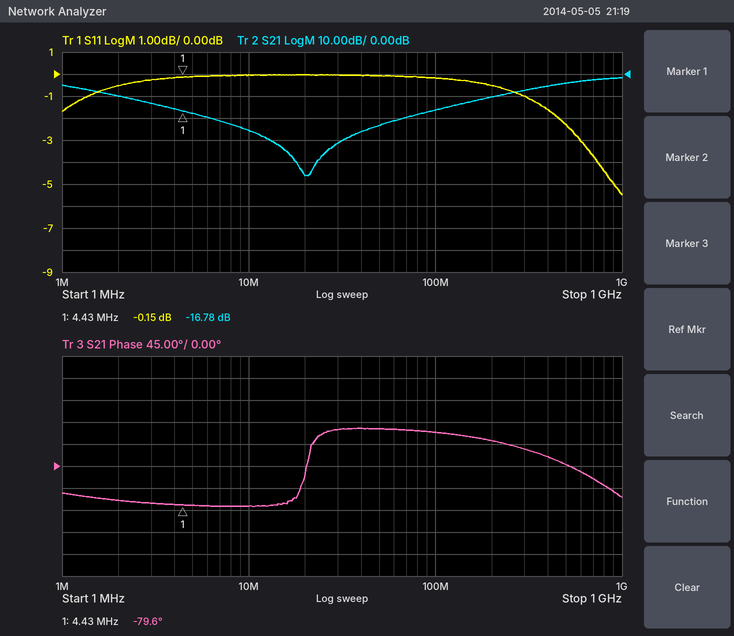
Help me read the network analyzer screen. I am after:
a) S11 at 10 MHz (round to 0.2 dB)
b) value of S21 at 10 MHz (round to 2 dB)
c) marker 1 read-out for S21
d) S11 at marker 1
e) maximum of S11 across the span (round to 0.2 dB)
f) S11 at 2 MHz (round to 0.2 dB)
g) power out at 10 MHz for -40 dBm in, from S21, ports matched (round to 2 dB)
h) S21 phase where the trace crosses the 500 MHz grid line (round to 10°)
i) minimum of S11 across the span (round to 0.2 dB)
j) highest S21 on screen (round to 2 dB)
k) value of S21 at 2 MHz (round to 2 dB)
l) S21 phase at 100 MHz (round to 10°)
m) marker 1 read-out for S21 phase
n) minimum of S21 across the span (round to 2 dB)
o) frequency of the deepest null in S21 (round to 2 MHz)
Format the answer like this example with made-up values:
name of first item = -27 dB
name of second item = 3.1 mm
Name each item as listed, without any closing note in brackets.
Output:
S11 at 10 MHz = 0.0 dB
value of S21 at 10 MHz = -26 dB
marker 1 read-out for S21 = -16.78 dB
S11 at marker 1 = -0.15 dB
maximum of S11 across the span = 0.0 dB
S11 at 2 MHz = -0.6 dB
power out at 10 MHz for -40 dBm in, from S21, ports matched = -66 dBm
S21 phase where the trace crosses the 500 MHz grid line = 0°
minimum of S11 across the span = -5.4 dB
highest S21 on screen = -2 dB
value of S21 at 2 MHz = -10 dB
S21 phase at 100 MHz = 70°
marker 1 read-out for S21 phase = -79.6°
minimum of S21 across the span = -46 dB
frequency of the deepest null in S21 = 20 MHz
